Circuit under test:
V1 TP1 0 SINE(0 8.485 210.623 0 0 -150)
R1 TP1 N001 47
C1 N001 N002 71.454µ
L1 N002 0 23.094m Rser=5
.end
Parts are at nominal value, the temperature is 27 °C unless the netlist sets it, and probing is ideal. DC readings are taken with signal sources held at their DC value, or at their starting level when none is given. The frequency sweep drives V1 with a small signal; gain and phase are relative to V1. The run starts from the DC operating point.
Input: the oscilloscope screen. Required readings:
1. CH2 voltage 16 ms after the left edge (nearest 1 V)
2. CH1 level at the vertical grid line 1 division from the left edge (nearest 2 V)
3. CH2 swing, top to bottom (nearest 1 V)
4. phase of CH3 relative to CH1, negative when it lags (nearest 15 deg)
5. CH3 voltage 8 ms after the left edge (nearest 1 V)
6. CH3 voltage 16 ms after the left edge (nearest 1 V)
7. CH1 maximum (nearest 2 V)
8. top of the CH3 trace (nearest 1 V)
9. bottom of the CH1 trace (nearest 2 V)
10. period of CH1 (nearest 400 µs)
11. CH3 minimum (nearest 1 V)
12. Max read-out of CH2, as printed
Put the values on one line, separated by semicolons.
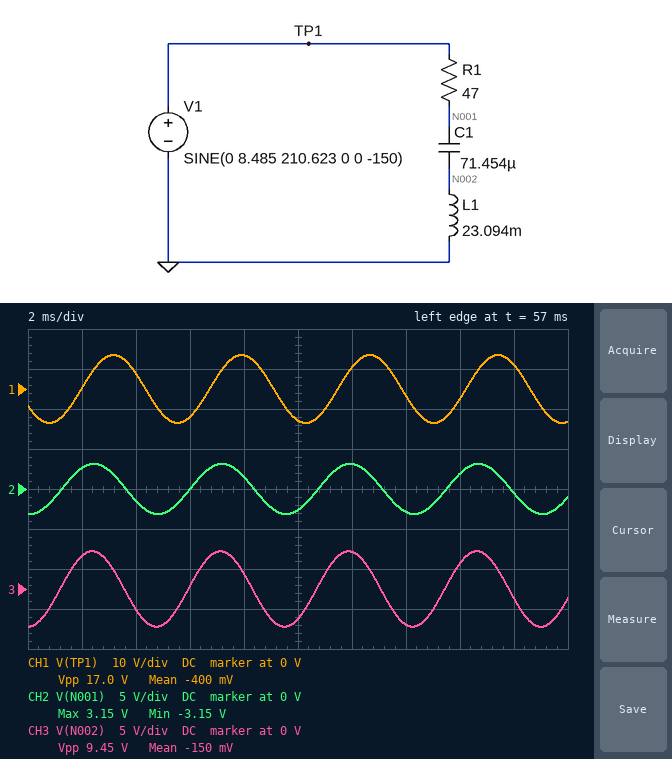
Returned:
2 V; 0 V; 6 V; 60 deg; 2 V; 3 V; 8 V; 5 V; -8 V; 4.8 ms; -5 V; 3.15 V
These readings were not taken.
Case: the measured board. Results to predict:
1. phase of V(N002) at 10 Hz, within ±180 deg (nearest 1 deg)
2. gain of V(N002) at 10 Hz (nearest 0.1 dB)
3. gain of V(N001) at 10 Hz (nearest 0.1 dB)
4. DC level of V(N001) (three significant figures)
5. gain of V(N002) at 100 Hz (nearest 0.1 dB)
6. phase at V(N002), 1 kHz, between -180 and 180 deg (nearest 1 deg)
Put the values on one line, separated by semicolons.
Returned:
93 deg; -32.8 dB; -0.2 dB; -4.24 V; -10.7 dB; 18 deg
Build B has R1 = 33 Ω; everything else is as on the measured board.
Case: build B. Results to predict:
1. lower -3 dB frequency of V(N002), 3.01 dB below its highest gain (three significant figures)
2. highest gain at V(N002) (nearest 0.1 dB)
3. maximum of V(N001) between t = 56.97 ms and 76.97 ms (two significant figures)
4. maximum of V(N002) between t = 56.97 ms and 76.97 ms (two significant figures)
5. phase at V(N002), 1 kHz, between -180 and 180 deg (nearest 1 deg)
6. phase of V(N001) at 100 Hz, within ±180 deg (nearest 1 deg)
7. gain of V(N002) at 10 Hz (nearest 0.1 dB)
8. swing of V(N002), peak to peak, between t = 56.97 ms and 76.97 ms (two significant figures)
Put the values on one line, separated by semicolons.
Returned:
203 Hz; 0 dB; 4.1 V; 6.1 V; 13 deg; -46 deg; -32.7 dB; 12 V
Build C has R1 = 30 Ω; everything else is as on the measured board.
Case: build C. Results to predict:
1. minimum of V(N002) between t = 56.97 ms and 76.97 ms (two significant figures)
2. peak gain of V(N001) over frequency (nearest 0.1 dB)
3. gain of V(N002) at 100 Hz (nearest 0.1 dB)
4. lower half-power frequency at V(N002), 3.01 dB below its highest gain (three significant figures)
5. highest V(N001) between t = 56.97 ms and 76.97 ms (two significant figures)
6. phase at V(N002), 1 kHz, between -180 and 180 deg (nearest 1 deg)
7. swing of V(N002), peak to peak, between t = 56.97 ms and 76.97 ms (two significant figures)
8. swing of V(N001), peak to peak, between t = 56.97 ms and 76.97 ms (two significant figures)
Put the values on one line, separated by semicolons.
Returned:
-6.5 V; 0 dB; -7.4 dB; 180 Hz; 4.3 V; 12 deg; 13 V; 8.7 V
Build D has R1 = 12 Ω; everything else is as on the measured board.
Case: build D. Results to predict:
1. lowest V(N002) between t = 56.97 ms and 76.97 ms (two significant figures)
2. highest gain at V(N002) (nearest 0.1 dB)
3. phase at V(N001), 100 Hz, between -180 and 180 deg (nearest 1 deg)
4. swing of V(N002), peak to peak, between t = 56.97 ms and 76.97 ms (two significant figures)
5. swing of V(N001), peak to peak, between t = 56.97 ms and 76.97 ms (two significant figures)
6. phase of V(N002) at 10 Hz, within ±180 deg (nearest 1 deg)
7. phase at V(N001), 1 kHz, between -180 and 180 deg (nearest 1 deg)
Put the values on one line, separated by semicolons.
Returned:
-10 V; 1.8 dB; -33 deg; 20 V; 13 V; 102 deg; 5 deg
